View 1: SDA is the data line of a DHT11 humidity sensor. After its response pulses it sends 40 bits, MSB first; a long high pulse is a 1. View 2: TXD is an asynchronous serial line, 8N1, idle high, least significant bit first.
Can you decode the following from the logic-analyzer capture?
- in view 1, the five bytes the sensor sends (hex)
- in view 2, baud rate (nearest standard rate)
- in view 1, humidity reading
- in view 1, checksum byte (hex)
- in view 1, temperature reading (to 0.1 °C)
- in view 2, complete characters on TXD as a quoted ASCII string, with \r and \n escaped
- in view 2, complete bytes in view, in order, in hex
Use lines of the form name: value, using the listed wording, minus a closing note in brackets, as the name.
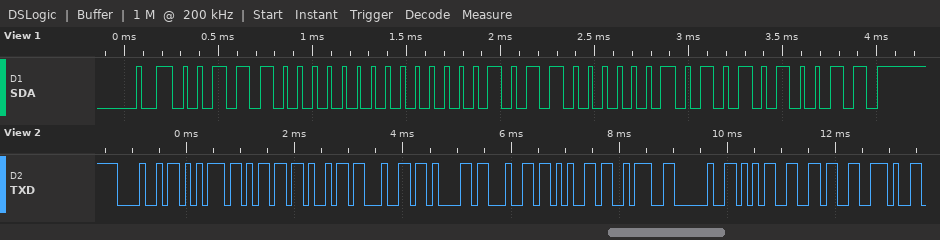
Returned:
in view 1, the five bytes the sensor sends: 38 00 16 05 53
in view 2, baud rate: 9600 baud
in view 1, humidity reading: 56 %
in view 1, checksum byte: 0x53
in view 1, temperature reading: 22.5 °C
in view 2, complete characters on TXD as a quoted ASCII string, with \r and \n escaped: "Humidade: 56."
in view 2, complete bytes in view, in order, in hex: 48 75 6D 69 64 61 64 65 3A 20 35 36 2E
